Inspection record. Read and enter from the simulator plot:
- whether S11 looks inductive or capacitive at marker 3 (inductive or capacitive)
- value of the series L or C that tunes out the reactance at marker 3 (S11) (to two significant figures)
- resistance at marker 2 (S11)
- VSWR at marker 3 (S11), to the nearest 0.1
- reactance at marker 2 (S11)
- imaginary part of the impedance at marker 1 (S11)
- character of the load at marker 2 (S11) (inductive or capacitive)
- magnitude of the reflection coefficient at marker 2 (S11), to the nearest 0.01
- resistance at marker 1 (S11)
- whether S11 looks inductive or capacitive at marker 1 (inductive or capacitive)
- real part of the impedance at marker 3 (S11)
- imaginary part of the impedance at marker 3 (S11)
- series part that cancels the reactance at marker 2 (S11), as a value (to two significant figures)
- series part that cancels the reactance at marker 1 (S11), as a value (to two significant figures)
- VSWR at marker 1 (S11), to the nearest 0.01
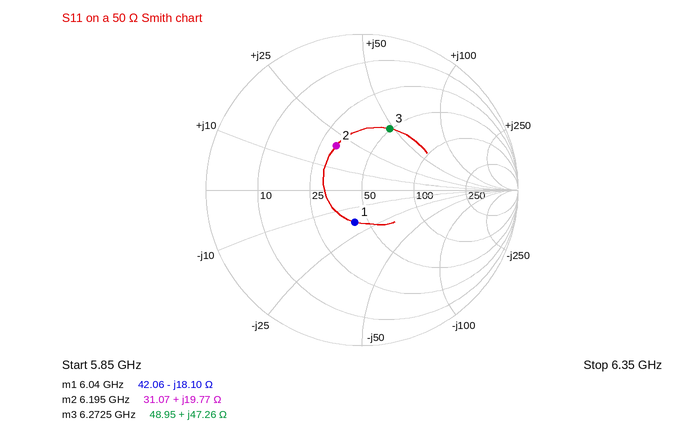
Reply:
inductive
540 fF
31.07 Ω
2.5
+19.77 Ω
-18.10 Ω
inductive
0.33
42.06 Ω
capacitive
48.95 Ω
+47.26 Ω
1.3 pF
480 pH
1.53
